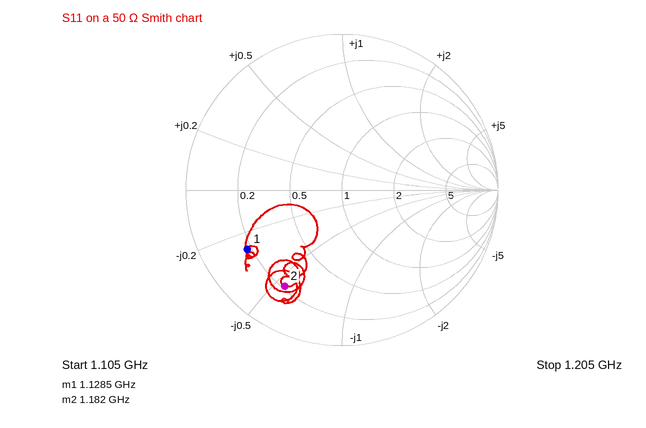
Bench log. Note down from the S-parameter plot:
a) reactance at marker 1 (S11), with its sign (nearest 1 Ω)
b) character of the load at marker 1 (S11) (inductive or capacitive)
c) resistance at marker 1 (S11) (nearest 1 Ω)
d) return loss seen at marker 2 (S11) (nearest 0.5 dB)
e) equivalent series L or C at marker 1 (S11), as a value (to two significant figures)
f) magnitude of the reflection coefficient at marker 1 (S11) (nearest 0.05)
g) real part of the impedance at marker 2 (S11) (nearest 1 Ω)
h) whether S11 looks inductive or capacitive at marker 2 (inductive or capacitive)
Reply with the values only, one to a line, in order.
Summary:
-14 Ω
capacitive
9 Ω
3.0 dB
10 pF
0.70
11 Ω
capacitive
